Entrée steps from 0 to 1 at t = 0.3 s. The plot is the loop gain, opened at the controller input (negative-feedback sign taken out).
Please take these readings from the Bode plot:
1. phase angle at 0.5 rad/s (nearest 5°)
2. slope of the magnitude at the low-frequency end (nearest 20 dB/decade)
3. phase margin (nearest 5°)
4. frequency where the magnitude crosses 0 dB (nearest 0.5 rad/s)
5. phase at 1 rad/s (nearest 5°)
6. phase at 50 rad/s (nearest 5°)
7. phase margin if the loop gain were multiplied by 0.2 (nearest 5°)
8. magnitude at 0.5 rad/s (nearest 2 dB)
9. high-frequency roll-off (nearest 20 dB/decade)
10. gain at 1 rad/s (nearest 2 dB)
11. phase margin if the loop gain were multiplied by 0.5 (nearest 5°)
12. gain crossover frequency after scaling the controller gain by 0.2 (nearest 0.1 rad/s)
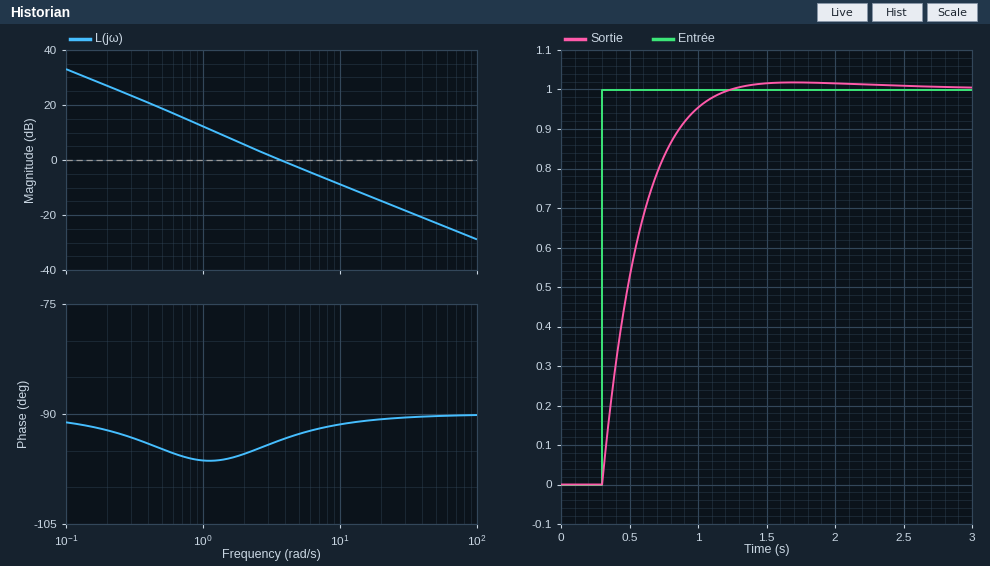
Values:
-95°
-20 dB/decade
85°
3.5 rad/s
-95°
-90°
85°
18 dB
-20 dB/decade
12 dB
85°
0.8 rad/s
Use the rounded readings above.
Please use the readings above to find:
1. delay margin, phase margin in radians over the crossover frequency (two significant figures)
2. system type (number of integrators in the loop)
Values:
0.42 s
1
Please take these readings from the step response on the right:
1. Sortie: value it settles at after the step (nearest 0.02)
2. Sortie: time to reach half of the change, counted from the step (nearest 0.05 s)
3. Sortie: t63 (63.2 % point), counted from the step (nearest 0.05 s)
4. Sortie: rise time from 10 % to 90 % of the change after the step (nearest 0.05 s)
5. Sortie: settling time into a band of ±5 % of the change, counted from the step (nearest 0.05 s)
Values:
1.00
0.20 s
0.25 s
0.55 s
0.70 s
